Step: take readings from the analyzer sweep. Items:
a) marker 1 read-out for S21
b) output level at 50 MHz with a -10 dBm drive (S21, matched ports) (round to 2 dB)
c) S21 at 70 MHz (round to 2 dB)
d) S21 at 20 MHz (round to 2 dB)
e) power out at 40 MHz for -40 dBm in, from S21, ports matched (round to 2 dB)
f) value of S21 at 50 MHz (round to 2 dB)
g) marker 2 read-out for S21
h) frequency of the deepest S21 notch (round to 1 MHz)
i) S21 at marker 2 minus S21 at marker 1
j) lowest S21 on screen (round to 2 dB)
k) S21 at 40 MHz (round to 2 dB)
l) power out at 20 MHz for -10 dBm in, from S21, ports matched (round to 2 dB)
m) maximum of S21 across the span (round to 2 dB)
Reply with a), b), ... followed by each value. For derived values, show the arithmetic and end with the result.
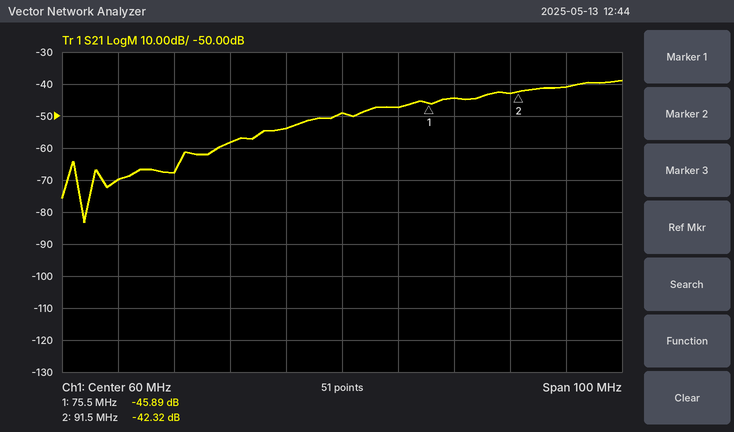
a) -45.89 dB
b) -10 dBm + (-54 dB) = -64 dBm
c) -48 dB
d) -70 dB
e) -40 dBm + (-58 dB) = -98 dBm
f) -54 dB
g) -42.32 dB
h) 14 MHz
i) -42.32 − (-45.89) = 3.57 dB
j) -84 dB
k) -58 dB
l) -10 dBm + (-70 dB) = -80 dBm
m) -38 dB
